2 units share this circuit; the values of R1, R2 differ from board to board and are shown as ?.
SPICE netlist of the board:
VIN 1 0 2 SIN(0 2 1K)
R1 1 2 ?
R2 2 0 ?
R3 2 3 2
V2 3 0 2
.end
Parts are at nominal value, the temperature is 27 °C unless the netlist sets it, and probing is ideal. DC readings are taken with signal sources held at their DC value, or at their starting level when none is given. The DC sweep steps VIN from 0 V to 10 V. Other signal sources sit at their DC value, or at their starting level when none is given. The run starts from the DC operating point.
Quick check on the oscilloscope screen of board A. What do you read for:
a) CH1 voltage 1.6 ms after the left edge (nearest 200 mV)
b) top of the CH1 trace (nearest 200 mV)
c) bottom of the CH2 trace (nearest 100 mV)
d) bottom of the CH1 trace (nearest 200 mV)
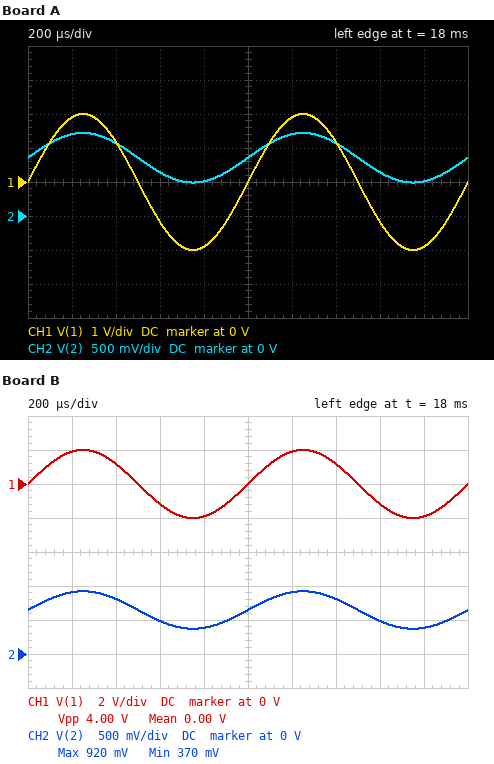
-1.2 V
2.0 V
500 mV
-2.0 V
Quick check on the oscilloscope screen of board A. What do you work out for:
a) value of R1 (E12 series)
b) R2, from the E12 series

4.7 Ω
2.2 Ω
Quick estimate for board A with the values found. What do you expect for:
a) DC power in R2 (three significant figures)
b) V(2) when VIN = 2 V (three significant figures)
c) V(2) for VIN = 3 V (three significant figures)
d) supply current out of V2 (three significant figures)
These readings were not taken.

678 mW
1.22 V
1.40 V
389 mA
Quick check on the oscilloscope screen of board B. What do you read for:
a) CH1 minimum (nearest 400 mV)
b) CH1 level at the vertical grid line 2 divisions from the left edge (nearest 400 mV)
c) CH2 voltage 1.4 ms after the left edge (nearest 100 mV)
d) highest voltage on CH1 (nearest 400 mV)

-2.0 V
1.2 V
800 mV
2.0 V
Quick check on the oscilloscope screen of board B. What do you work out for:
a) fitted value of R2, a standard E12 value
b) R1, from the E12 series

1.2 Ω
4.7 Ω
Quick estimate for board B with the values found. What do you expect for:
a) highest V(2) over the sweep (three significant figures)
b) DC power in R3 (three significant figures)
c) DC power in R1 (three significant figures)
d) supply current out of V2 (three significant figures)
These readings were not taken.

2.02 V
581 mW
247 mW
539 mA
